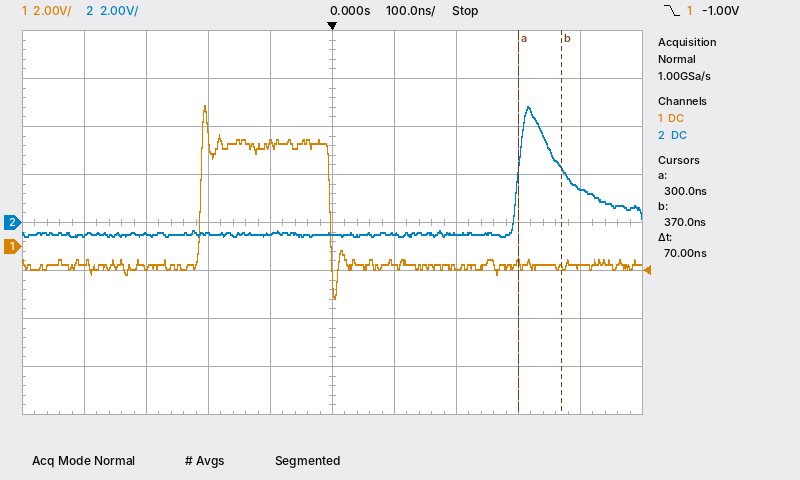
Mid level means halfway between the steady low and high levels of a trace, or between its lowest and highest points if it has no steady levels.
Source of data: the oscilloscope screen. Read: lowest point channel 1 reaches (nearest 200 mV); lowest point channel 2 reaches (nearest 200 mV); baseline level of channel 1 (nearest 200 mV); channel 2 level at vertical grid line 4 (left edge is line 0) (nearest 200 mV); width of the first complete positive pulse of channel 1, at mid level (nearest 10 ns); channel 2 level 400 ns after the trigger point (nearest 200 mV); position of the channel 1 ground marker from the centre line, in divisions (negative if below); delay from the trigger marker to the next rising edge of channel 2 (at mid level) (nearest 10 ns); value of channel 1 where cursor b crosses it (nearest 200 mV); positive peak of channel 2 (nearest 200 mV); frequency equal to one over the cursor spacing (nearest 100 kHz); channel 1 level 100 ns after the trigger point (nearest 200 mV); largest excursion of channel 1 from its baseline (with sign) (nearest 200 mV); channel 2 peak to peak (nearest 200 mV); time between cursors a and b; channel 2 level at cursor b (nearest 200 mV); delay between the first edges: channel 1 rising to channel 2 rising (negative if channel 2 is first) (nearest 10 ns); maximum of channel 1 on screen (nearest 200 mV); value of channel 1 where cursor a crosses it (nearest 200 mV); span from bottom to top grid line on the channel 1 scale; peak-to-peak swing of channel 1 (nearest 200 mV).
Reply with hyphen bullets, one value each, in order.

- -2.2 V
- -600 mV
- -800 mV
- -400 mV
- 210 ns
- 1.4 V
- -0.5 div
- 300 ns
- -800 mV
- 4.8 V
- 14.3 MHz
- -600 mV
- +6.6 V
- 5.4 V
- 70 ns
- 2.2 V
- +510 ns
- 5.8 V
- -800 mV
- 16 V
- 8.0 V
